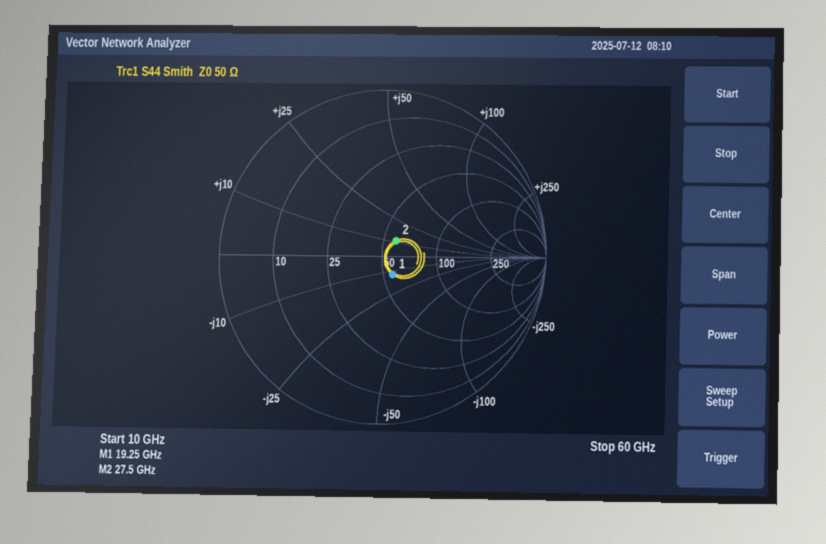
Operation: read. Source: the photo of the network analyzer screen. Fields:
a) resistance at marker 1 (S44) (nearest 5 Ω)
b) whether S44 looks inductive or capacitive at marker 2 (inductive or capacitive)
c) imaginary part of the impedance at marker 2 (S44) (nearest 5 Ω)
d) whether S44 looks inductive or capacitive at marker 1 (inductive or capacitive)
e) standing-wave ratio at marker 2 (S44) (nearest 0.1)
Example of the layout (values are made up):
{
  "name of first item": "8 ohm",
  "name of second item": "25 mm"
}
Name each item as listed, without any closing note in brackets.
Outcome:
{
  "resistance at marker 1 (S44)": "55 Ω",
  "whether S44 looks inductive or capacitive at marker 2": "inductive",
  "imaginary part of the impedance at marker 2 (S44)": "+10 Ω",
  "whether S44 looks inductive or capacitive at marker 1": "capacitive",
  "standing-wave ratio at marker 2 (S44)": "1.3"
}
